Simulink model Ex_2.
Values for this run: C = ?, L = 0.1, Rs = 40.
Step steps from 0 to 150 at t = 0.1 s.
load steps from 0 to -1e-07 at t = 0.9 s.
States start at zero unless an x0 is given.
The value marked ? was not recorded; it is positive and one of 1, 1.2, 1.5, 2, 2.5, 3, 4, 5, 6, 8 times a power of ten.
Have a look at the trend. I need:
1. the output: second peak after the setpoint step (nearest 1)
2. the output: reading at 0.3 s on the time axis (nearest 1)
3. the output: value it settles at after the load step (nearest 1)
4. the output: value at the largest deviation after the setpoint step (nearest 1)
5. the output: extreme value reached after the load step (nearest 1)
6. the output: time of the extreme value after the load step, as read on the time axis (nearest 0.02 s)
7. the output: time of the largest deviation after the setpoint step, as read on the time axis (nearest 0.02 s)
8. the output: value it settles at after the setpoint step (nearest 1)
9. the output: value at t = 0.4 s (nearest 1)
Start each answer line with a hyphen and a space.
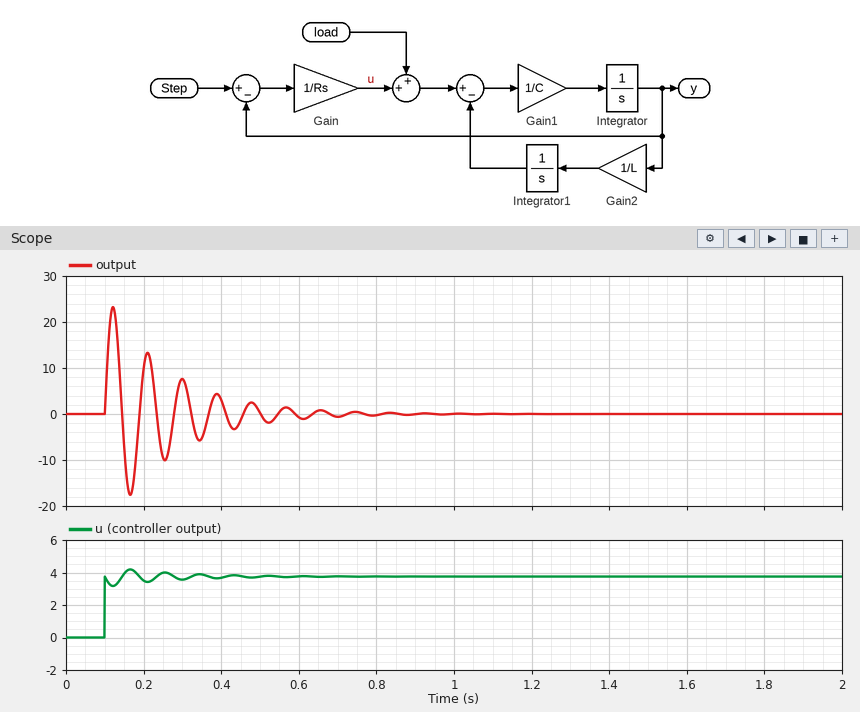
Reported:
- 13
- 8
- 0
- 23
- 0
- 0.92 s
- 0.12 s
- 0
- 3
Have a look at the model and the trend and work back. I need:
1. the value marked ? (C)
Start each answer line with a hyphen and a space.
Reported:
- 0.002
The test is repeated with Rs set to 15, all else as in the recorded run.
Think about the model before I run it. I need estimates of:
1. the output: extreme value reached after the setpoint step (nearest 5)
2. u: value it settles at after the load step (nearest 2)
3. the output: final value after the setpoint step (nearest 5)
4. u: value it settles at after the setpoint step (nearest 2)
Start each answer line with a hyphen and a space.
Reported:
- 50
- 10
- 0
- 10
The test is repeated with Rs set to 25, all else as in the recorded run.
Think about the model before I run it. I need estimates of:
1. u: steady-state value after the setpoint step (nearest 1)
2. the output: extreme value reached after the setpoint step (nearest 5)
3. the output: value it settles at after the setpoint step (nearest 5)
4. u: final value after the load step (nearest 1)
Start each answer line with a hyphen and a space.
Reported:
- 6
- 35
- 0
- 6
